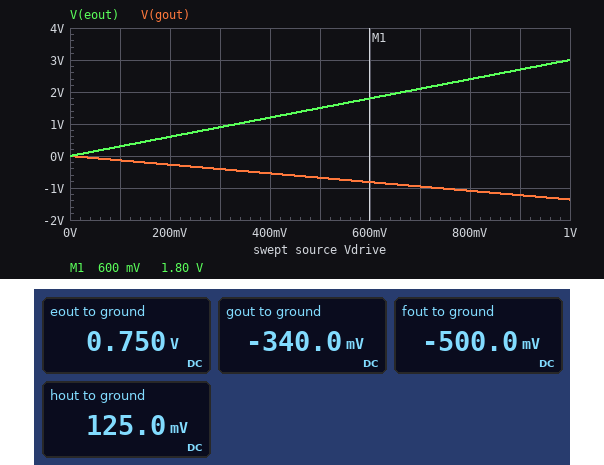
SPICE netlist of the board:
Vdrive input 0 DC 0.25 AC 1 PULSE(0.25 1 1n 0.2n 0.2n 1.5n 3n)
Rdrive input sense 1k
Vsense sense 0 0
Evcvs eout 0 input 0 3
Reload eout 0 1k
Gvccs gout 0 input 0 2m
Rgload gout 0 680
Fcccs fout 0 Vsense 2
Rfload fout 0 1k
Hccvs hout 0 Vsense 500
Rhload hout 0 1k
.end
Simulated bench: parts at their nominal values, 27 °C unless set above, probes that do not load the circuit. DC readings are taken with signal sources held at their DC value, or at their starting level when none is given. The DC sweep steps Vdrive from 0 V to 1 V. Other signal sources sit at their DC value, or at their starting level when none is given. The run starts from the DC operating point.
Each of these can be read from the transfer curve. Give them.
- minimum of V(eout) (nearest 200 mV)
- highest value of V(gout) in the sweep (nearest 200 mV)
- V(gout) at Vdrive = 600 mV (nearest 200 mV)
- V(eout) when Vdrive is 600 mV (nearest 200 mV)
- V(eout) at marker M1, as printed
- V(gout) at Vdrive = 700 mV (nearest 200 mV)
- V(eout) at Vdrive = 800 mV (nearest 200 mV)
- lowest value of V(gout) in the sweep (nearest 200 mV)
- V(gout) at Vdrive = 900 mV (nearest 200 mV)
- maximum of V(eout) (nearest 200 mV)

0 V
0 V
-800 mV
1.8 V
1.80 V
-1.0 V
2.4 V
-1.4 V
-1.2 V
3.0 V
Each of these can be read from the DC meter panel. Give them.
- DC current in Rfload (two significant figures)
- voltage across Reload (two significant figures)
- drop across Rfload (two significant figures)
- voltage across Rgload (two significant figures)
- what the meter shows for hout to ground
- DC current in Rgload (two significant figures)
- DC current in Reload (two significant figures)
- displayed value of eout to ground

500 µA
750 mV
500 mV
340 mV
125.0 mV
500 µA
750 µA
0.750 V
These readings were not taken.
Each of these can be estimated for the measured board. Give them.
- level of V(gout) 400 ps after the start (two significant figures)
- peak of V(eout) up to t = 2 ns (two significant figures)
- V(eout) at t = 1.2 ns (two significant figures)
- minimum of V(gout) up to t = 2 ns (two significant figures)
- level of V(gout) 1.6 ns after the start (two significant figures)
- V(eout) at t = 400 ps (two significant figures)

-340 mV
3.0 V
3.0 V
-1.4 V
-1.4 V
750 mV
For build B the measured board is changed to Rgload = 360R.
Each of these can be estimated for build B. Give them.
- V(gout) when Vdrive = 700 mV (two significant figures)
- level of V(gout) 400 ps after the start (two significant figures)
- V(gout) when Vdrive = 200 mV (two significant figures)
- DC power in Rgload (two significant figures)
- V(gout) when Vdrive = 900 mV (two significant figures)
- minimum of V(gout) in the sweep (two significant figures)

-500 mV
-180 mV
-140 mV
90 µW
-650 mV
-720 mV
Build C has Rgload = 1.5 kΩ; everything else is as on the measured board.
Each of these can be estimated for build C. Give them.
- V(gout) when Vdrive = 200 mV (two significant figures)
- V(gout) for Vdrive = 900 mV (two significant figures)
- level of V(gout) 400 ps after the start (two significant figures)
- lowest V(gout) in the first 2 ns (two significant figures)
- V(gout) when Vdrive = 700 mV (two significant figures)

-600 mV
-2.7 V
-750 mV
-3.0 V
-2.1 V
